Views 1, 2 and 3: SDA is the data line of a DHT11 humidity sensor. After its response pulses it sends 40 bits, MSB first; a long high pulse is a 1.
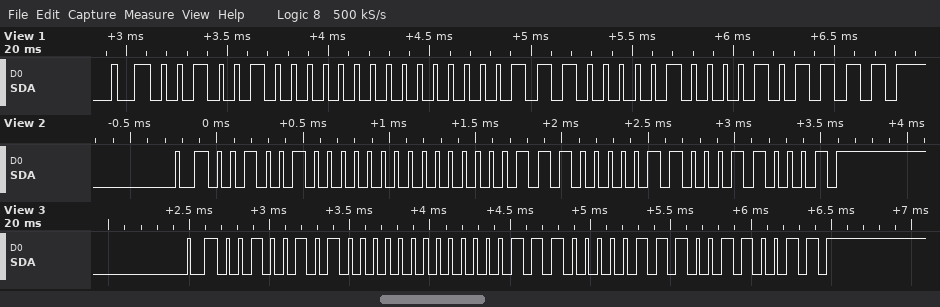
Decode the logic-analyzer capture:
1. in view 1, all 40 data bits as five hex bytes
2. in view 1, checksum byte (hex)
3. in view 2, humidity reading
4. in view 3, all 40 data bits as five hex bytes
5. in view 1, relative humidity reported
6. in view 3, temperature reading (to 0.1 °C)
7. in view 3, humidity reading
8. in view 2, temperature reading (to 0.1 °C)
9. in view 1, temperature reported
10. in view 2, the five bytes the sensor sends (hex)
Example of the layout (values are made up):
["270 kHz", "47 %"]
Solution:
["24 00 07 04 2F", "0x2F", "36 %", "25 00 07 07 33", "36 %", "7.7 °C", "37 %", "7.6 °C", "7.4 °C", "24 00 07 06 31"]
